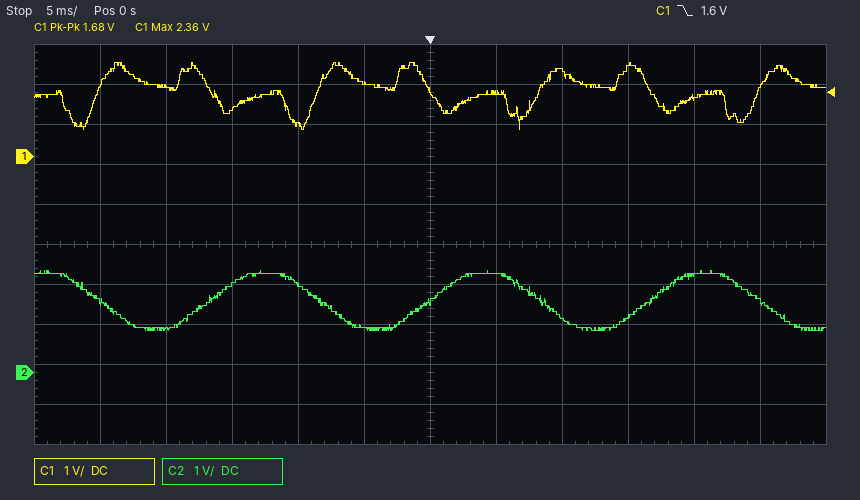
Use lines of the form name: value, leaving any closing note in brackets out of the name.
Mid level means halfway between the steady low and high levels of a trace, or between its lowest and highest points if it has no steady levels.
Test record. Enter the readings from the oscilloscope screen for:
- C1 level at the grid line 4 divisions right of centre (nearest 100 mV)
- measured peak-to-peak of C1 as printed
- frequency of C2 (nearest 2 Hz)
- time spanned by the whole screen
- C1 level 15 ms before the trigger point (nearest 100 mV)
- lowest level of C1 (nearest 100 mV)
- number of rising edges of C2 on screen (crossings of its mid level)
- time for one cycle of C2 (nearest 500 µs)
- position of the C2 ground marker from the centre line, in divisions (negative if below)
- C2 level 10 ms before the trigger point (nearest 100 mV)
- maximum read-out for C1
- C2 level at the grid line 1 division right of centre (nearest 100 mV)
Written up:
C1 level at the grid line 4 divisions right of centre: 1.5 V
measured peak-to-peak of C1 as printed: 1.68 V
frequency of C2: 60 Hz
time spanned by the whole screen: 60 ms
C1 level 15 ms before the trigger point: 1.2 V
lowest level of C1: 700 mV
number of rising edges of C2 on screen: 3
time for one cycle of C2: 16.5 ms
position of the C2 ground marker from the centre line, in divisions: -3.2 div
C2 level 10 ms before the trigger point: 2.2 V
maximum read-out for C1: 2.36 V
C2 level at the grid line 1 division right of centre: 2.5 V
